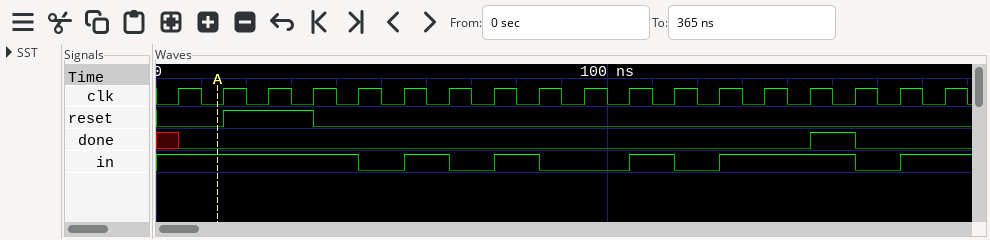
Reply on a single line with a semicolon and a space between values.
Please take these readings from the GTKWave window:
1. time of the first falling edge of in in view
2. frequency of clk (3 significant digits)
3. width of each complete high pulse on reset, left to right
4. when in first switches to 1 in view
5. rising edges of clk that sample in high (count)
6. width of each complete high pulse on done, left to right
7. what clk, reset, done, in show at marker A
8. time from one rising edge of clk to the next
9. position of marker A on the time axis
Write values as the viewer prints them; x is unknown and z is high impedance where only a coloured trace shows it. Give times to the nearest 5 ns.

45 ns; 100 MHz; 20 ns; 55 ns; 12; 10 ns; clk=0, reset=0, done=0, in=1; 10 ns; 15 ns
